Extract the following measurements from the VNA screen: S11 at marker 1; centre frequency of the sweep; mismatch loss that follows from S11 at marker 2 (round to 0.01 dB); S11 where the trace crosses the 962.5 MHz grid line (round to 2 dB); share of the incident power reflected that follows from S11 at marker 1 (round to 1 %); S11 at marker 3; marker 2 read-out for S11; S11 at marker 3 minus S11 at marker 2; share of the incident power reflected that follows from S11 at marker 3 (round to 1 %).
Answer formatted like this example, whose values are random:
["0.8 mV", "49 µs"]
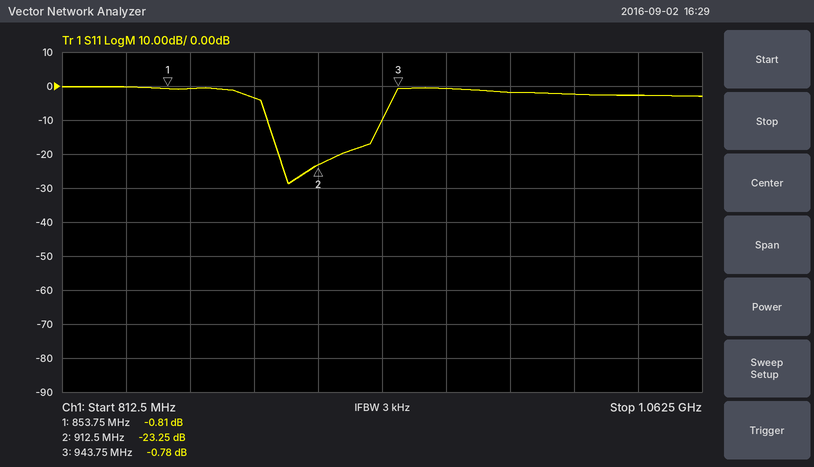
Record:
["-0.81 dB", "937.5 MHz", "0.02 dB", "0 dB", "83 %", "-0.78 dB", "-23.25 dB", "22.47 dB", "84 %"]
